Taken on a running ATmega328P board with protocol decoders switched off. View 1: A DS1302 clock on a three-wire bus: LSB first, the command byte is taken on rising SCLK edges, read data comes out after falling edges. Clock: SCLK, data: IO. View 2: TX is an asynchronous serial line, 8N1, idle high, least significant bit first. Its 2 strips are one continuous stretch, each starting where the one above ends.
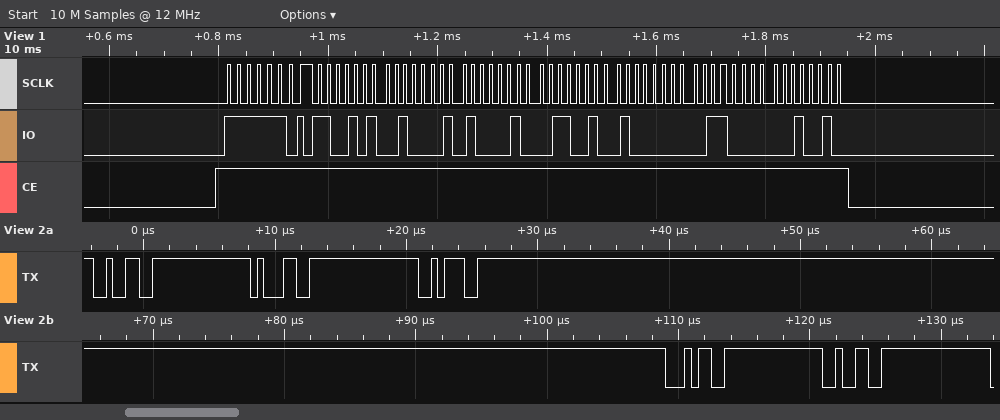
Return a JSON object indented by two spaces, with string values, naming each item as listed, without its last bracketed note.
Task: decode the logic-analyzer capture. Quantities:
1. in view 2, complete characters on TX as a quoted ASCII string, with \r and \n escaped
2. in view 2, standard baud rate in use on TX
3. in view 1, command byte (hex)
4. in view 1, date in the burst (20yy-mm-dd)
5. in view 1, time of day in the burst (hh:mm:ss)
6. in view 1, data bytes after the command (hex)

{
  "in view 2, complete characters on TX as a quoted ASCII string, with \\r and \\n escaped": "\"21:42\"",
  "in view 2, standard baud rate in use on TX": "2000000 baud",
  "in view 1, command byte": "0xBF",
  "in view 1, date in the burst": "2024-01-26",
  "in view 1, time of day in the burst": "21:42:53",
  "in view 1, data bytes after the command": "53 42 21 26 01 06 24"
}
